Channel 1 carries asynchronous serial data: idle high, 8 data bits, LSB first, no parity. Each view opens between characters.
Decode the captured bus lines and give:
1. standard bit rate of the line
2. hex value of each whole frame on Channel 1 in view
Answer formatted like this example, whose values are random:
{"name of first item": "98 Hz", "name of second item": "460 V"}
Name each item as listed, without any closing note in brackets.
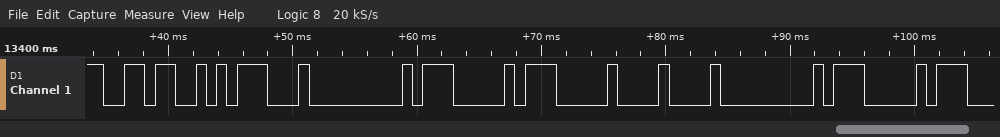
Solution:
{"standard bit rate of the line": "1200 baud", "hex value of each whole frame on Channel 1 in view": "36, 1D, 00, 07, 07, 08, 00, 07"}
